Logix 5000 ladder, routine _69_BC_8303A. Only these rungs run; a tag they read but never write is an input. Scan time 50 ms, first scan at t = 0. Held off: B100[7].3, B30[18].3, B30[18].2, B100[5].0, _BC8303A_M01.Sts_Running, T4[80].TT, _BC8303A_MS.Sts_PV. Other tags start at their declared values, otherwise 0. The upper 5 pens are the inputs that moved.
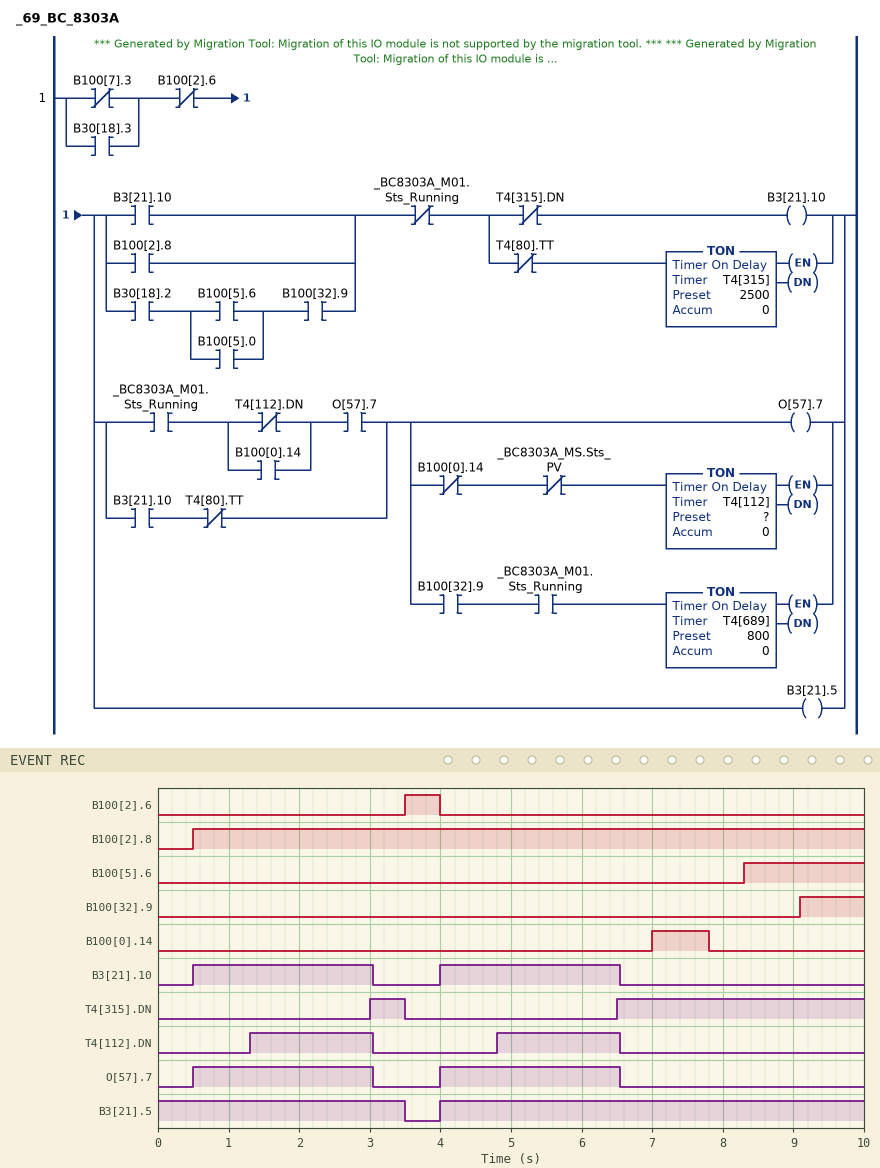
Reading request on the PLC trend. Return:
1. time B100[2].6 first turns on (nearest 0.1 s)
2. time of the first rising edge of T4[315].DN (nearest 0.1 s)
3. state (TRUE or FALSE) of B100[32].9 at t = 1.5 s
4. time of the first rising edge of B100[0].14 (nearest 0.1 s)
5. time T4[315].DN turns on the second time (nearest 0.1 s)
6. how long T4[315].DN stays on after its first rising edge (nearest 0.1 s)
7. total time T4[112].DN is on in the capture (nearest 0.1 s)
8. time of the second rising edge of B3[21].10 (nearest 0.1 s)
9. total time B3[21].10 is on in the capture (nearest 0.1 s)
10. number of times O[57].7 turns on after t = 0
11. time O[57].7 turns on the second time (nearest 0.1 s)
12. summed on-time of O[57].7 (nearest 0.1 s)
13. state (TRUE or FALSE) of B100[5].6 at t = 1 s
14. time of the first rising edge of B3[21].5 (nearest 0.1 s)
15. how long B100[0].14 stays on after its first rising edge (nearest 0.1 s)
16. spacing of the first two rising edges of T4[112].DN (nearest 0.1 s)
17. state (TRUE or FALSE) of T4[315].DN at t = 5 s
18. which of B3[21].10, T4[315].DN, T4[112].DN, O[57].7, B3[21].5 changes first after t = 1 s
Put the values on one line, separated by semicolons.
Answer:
3.5 s; 3.0 s; FALSE; 7.0 s; 6.5 s; 0.5 s; 3.5 s; 4.0 s; 5.1 s; 2; 4.0 s; 5.1 s; FALSE; 4.0 s; 0.8 s; 3.5 s; FALSE; T4[112].DN
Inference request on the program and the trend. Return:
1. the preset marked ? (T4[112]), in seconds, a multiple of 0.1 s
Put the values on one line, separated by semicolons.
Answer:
0.8 s
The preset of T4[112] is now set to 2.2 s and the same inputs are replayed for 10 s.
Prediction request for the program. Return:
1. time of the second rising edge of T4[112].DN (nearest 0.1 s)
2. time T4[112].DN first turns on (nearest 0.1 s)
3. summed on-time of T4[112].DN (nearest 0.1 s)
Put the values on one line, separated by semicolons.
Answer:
6.2 s; 2.7 s; 0.7 s
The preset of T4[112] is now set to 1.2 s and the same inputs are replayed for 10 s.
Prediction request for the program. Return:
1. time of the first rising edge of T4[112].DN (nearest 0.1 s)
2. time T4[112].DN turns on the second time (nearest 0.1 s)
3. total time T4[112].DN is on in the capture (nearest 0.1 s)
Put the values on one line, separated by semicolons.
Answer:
1.7 s; 5.2 s; 2.7 s
